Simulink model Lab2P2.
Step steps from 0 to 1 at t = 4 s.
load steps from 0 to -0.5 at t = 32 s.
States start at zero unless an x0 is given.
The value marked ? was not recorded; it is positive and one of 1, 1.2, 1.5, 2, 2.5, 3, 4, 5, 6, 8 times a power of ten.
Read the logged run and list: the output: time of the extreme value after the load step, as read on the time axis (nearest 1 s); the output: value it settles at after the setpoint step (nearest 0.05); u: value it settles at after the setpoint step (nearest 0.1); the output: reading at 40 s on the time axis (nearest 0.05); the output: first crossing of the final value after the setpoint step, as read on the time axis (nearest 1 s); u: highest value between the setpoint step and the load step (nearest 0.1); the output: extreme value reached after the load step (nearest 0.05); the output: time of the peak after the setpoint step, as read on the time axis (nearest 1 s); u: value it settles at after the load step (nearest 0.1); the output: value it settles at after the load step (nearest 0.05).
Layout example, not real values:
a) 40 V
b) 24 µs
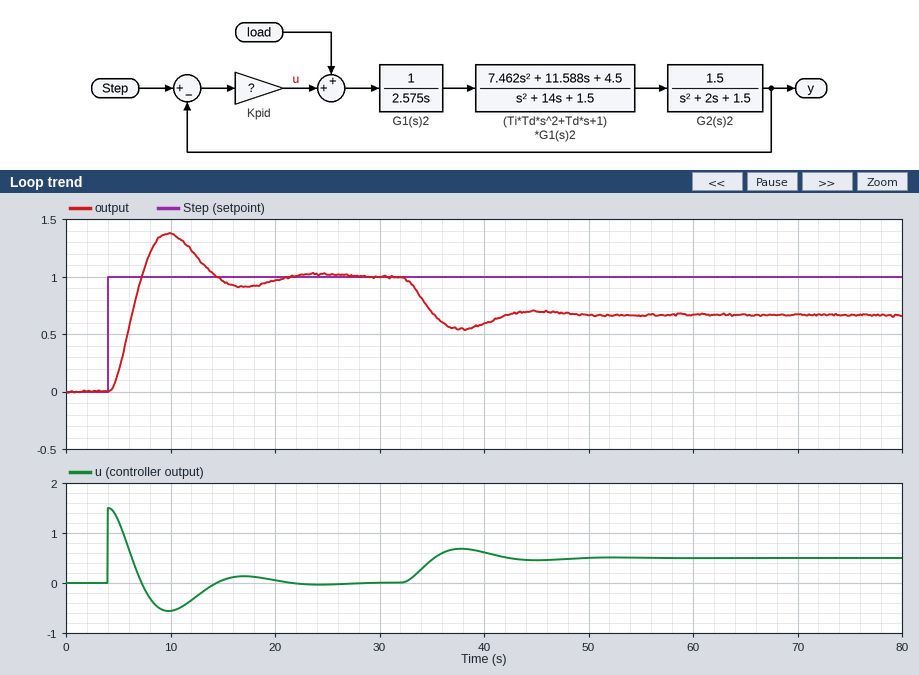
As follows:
a) 38 s
b) 1.00
c) 0.0
d) 0.60
e) 7 s
f) 1.5
g) 0.55
h) 10 s
i) 0.5
j) 0.65
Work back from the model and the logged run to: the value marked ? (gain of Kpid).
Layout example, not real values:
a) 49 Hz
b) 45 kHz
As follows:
a) 1.5
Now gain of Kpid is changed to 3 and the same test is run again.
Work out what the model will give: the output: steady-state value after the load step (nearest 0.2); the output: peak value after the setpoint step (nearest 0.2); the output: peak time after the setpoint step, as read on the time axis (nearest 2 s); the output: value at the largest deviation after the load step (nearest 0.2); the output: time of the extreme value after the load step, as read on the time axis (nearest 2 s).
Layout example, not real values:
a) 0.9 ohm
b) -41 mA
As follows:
a) 0.8
b) 1.4
c) 8 s
d) 0.8
e) 36 s
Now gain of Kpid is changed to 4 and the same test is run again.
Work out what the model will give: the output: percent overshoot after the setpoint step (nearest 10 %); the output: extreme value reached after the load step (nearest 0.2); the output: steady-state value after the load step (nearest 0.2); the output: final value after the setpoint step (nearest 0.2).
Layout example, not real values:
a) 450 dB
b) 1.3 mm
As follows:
a) 50 %
b) 0.8
c) 0.8
d) 1.0
